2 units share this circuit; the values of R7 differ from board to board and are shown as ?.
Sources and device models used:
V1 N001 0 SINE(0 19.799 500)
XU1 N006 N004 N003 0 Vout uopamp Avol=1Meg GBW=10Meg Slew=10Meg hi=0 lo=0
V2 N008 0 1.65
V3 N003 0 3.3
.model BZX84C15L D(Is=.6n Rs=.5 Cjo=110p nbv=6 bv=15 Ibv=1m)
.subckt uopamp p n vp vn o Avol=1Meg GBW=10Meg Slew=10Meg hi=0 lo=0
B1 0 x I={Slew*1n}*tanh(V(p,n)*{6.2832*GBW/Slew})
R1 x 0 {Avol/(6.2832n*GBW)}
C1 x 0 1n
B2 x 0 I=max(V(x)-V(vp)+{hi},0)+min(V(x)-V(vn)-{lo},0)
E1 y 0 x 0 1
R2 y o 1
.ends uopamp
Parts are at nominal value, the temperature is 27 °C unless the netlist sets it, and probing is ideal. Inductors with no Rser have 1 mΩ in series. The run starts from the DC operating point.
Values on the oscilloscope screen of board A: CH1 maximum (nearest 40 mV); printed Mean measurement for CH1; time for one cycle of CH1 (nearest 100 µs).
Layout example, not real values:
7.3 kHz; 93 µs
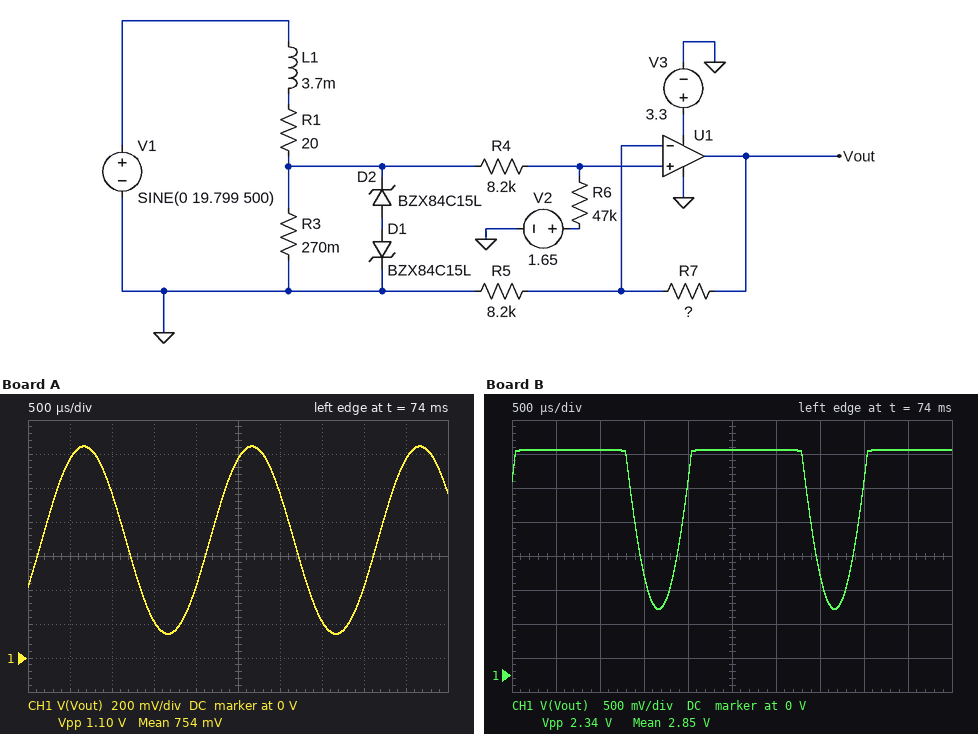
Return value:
1.24 V; 754 mV; 2.0 ms
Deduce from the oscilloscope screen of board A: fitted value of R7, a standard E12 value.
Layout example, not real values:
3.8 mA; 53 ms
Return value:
15 kΩ
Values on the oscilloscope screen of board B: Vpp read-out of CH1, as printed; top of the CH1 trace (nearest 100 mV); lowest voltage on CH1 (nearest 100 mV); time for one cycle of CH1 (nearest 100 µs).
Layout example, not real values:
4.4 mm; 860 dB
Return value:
2.34 V; 3.3 V; 1.0 V; 2.0 ms
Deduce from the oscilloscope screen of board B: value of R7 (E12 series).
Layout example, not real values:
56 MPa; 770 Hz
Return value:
150 kΩ
